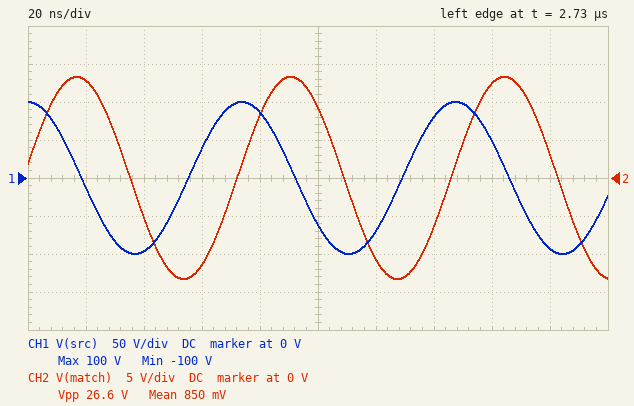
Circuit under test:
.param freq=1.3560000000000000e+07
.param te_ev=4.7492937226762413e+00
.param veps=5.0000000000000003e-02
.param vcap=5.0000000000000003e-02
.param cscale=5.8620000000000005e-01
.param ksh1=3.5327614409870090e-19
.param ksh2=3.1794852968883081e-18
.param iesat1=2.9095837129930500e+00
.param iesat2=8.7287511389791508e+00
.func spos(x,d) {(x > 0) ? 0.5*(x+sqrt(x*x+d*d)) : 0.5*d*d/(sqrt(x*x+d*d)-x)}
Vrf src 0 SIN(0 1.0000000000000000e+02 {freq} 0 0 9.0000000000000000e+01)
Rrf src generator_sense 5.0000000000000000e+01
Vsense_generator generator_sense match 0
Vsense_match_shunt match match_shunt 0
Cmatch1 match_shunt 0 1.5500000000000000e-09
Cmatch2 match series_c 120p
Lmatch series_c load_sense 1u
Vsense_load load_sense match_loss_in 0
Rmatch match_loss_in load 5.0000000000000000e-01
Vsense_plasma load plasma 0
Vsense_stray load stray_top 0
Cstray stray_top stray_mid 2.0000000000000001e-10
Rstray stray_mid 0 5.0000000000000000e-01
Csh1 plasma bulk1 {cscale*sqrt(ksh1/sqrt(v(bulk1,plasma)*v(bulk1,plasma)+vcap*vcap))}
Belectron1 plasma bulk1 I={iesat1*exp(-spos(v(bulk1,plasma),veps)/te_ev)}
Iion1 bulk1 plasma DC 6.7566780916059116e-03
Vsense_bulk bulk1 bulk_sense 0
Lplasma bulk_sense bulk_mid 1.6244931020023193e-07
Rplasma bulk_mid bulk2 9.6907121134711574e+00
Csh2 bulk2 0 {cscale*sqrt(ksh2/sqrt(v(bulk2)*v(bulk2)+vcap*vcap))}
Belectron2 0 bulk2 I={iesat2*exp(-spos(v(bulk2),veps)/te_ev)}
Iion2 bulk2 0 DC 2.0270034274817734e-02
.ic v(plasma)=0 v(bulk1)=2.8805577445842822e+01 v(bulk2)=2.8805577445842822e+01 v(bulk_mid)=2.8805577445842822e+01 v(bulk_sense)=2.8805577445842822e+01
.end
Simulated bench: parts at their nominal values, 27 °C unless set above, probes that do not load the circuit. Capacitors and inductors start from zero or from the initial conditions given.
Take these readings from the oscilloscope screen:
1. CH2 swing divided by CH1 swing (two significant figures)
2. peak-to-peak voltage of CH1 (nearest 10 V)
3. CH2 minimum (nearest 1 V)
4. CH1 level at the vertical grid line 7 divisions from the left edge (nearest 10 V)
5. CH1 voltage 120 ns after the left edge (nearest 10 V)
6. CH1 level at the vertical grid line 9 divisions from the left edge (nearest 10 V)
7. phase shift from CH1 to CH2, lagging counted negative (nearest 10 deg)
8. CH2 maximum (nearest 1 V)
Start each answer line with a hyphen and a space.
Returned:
- 0.13
- 200 V
- -13 V
- 80 V
- -70 V
- -90 V
- -80 deg
- 13 V
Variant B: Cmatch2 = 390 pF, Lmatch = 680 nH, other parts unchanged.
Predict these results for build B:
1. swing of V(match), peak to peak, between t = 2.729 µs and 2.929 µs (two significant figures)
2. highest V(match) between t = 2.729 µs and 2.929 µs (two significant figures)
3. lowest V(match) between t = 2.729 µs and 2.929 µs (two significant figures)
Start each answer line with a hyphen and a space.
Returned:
- 22 V
- 11 V
- -11 V
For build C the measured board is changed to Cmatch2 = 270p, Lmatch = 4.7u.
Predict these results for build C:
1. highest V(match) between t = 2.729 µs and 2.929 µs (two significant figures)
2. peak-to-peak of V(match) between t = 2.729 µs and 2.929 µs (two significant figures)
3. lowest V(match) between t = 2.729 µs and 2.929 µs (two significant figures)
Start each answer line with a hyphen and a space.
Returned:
- 15 V
- 31 V
- -15 V
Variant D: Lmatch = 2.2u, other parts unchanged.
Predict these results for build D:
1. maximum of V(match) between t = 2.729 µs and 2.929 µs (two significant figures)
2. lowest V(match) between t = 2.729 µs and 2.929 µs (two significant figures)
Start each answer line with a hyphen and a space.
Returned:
- 18 V
- -18 V
